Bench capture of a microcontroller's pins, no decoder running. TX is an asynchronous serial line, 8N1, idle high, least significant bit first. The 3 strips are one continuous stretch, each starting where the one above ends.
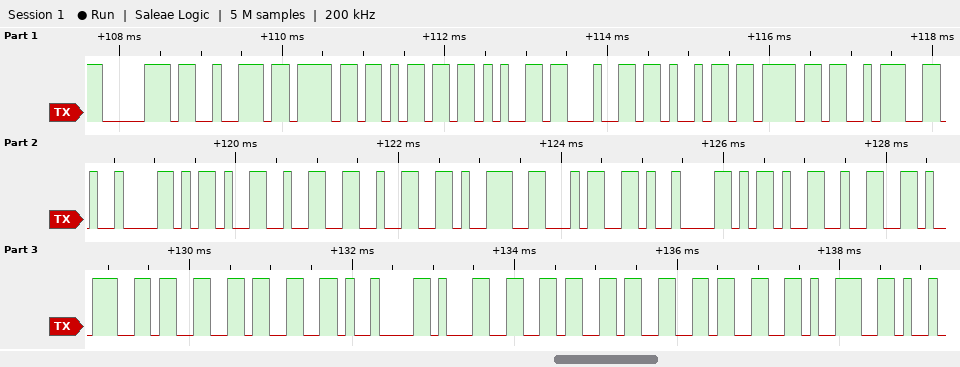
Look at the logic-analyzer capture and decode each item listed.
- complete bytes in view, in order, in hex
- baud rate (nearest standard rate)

70 72 6F 6D 65 64 69 6F 3A 09 2D 32 32 39 34 09 2D 32 39 33 33 09 31 36 33 33 39
9600 baud
